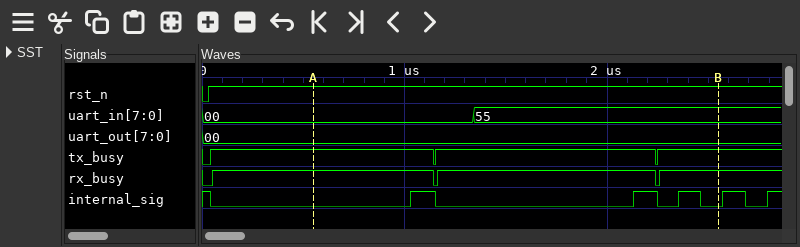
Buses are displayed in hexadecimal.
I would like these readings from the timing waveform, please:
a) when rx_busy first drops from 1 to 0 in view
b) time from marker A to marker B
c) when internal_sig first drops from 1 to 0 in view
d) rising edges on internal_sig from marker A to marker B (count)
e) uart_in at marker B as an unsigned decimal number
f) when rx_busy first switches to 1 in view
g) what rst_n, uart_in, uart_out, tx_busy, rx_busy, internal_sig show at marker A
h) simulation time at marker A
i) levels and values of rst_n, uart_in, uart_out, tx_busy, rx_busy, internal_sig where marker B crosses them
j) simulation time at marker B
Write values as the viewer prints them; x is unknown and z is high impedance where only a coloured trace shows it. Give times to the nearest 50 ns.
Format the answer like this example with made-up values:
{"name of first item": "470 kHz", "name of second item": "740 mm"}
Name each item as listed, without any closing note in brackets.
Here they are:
{"when rx_busy first drops from 1 to 0 in view": "1150 ns", "time from marker A to marker B": "2000 ns", "when internal_sig first drops from 1 to 0 in view": "50 ns", "rising edges on internal_sig from marker A to marker B": "3", "uart_in at marker B as an unsigned decimal number": "85", "when rx_busy first switches to 1 in view": "50 ns", "what rst_n, uart_in, uart_out, tx_busy, rx_busy, internal_sig show at marker A": "rst_n=1, uart_in=00, uart_out=00, tx_busy=1, rx_busy=1, internal_sig=0", "simulation time at marker A": "550 ns", "levels and values of rst_n, uart_in, uart_out, tx_busy, rx_busy, internal_sig where marker B crosses them": "rst_n=1, uart_in=55, uart_out=00, tx_busy=1, rx_busy=1, internal_sig=0", "simulation time at marker B": "2550 ns"}
